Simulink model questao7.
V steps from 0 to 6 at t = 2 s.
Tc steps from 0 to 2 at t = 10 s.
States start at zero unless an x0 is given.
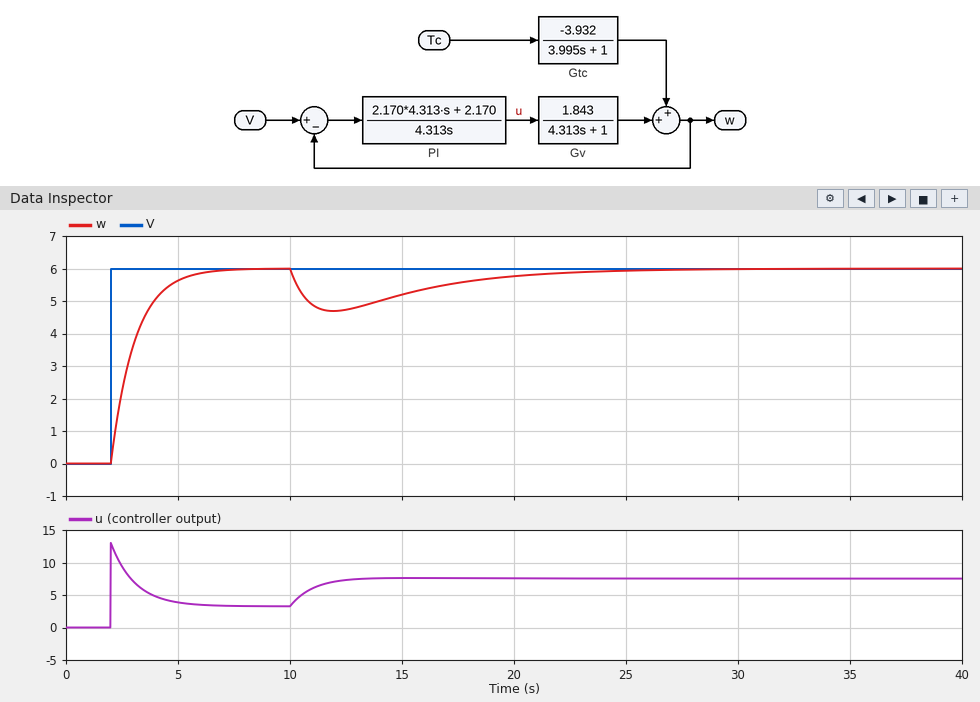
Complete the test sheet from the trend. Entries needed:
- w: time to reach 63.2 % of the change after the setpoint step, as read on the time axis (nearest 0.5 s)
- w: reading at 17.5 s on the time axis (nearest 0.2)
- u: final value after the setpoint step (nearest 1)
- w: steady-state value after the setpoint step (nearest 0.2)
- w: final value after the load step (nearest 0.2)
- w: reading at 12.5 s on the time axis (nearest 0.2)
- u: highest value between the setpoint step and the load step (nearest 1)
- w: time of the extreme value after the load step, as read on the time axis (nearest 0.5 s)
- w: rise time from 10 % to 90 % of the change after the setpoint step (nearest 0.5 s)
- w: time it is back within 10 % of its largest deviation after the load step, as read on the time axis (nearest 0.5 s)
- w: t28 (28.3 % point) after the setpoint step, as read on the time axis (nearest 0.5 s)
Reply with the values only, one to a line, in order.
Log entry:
3.0 s
5.6
3
6.0
6.0
4.8
13
12.0 s
2.5 s
22.5 s
2.5 s
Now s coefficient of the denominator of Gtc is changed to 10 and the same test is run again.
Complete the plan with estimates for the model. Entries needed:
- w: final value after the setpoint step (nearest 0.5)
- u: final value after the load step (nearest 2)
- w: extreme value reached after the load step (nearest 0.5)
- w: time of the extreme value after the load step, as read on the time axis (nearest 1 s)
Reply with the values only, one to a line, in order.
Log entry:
6.0
8
5.5
13 s
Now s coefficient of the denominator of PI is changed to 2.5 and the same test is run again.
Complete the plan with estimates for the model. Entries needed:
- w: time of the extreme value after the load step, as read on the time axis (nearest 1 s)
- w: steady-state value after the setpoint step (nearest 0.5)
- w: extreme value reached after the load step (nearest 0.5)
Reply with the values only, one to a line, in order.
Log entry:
11 s
6.0
5.0
